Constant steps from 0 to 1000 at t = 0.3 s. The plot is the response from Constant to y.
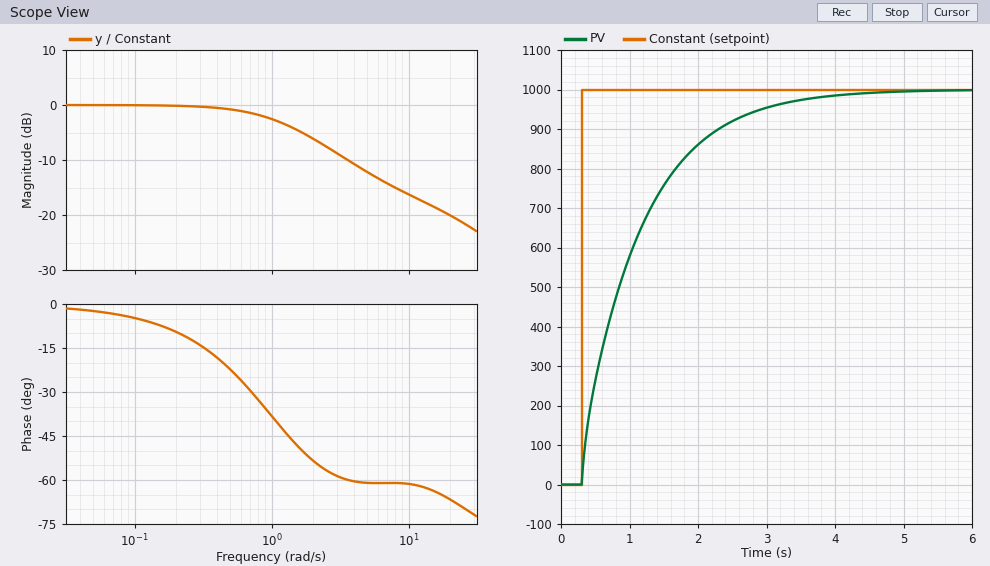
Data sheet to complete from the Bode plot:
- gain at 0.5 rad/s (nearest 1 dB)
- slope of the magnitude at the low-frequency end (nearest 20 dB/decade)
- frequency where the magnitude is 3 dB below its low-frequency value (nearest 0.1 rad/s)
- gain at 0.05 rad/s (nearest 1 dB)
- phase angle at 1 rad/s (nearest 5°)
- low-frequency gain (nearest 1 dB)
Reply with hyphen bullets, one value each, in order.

- -1 dB
- 0 dB/decade
- 1.1 rad/s
- 0 dB
- -40°
- 0 dB
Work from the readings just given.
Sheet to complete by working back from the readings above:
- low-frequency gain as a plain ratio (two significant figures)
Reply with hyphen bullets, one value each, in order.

- 1.0
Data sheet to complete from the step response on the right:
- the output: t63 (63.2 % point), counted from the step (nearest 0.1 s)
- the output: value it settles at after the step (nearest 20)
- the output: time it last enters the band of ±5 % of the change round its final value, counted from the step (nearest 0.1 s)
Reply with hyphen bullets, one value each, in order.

- 0.8 s
- 1000
- 2.6 s
